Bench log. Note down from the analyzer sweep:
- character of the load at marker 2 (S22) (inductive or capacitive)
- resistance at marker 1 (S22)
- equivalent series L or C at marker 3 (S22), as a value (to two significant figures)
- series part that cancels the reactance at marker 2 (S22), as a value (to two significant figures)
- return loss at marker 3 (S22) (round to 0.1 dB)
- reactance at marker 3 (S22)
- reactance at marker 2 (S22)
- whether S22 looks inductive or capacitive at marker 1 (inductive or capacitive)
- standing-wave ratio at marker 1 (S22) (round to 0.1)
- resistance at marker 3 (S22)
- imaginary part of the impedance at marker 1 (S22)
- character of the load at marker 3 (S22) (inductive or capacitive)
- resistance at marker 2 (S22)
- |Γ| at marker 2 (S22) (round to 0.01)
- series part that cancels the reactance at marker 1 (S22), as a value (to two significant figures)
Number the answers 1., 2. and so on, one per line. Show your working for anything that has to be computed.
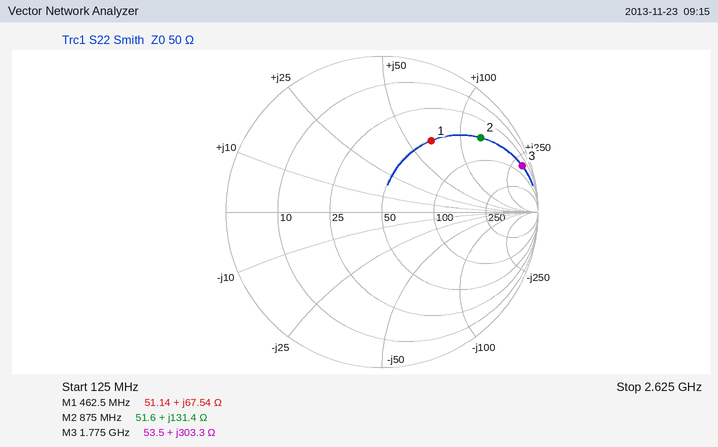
1. inductive
2. 51.14 Ω
3. L = 303.3 Ω/(2π × 1.775 GHz) ≈ 27 nH
4. C = 1/(2π × 875 MHz × 131.4 Ω) ≈ 1.4 pF
5. 0.5 dB
6. +303.3 Ω
7. +131.4 Ω
8. inductive
9. 3.5
10. 53.5 Ω
11. +67.54 Ω
12. inductive
13. 51.6 Ω
14. 0.79
15. C = 1/(2π × 462.5 MHz × 67.54 Ω) ≈ 5.1 pF
